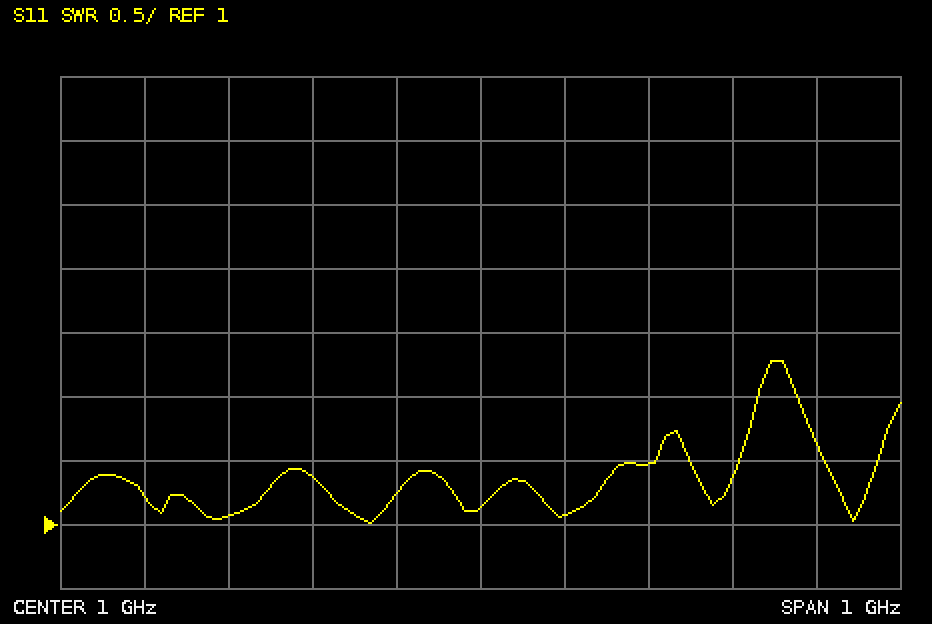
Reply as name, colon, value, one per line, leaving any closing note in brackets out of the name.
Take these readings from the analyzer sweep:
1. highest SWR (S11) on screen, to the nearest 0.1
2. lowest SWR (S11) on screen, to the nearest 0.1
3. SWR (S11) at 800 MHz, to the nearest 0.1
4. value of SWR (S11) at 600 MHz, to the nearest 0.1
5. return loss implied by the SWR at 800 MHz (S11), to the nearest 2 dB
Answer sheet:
highest SWR (S11) on screen, to the nearest 0.1: 2.3
lowest SWR (S11) on screen, to the nearest 0.1: 1.0
SWR (S11) at 800 MHz, to the nearest 0.1: 1.4
value of SWR (S11) at 600 MHz, to the nearest 0.1: 1.2
return loss implied by the SWR at 800 MHz (S11), to the nearest 2 dB: 16 dB
